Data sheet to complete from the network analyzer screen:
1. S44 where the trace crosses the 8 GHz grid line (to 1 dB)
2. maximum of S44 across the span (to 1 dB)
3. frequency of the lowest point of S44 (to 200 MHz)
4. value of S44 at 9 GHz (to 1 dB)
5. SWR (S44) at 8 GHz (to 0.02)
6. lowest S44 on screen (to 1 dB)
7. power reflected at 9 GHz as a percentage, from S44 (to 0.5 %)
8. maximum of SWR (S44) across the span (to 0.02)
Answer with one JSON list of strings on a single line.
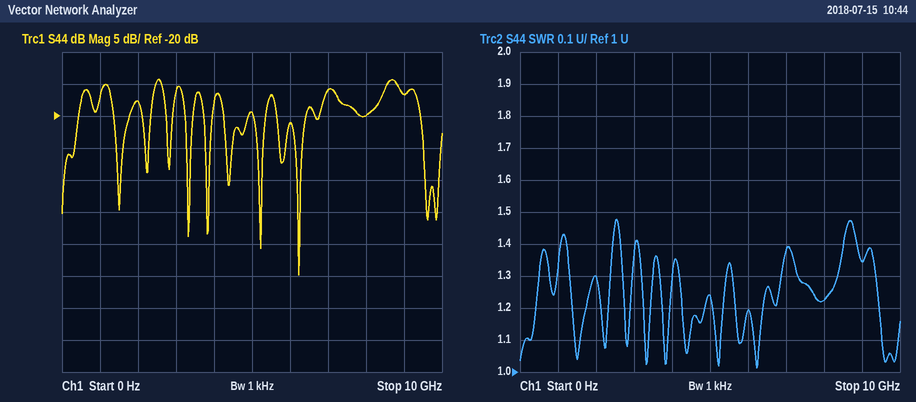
["-20 dB", "-14 dB", "6.2 GHz", "-17 dB", "1.22", "-45 dB", "2.0 %", "1.48"]
